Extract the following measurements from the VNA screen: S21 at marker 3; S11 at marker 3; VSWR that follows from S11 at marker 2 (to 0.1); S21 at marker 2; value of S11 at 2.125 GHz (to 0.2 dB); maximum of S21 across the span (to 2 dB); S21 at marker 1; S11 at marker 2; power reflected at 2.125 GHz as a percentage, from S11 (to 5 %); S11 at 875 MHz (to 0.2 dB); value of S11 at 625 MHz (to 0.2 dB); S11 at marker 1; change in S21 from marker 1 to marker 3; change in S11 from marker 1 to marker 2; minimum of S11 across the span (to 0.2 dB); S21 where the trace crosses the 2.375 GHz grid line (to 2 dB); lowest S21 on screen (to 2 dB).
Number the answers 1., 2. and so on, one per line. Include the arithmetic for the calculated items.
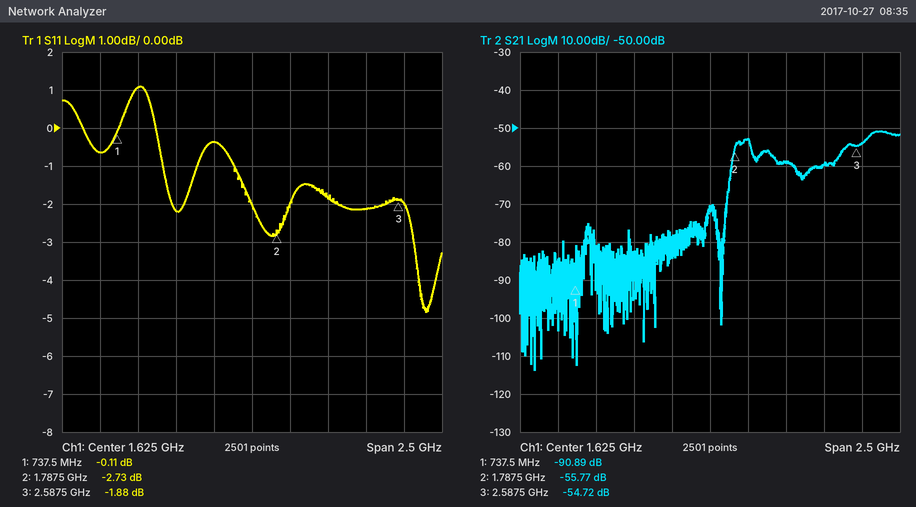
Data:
1. -54.72 dB
2. -1.88 dB
3. (1 + 0.7303)/(1 − 0.7303) ≈ 6.4
4. -55.77 dB
5. -1.8 dB
6. -50 dB
7. -90.89 dB
8. -2.73 dB
9. 10^(-1.8/10) ≈ 66.1 %, so 65 % to the nearest 5 %
10. 1.0 dB
11. -0.6 dB
12. -0.11 dB
13. -54.72 − (-90.89) = 36.17 dB
14. -2.73 − (-0.11) = -2.62 dB
15. -4.8 dB
16. -60 dB
17. -114 dB
